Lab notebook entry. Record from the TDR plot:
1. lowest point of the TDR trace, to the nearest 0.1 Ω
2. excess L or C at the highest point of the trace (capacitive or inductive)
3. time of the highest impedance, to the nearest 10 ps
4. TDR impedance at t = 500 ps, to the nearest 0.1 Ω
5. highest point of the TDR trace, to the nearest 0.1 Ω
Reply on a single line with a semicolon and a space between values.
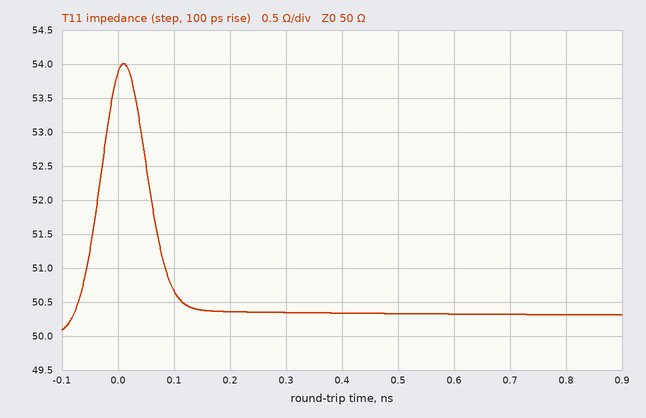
50.1 Ω; inductive; 10 ps; 50.3 Ω; 54.0 Ω
